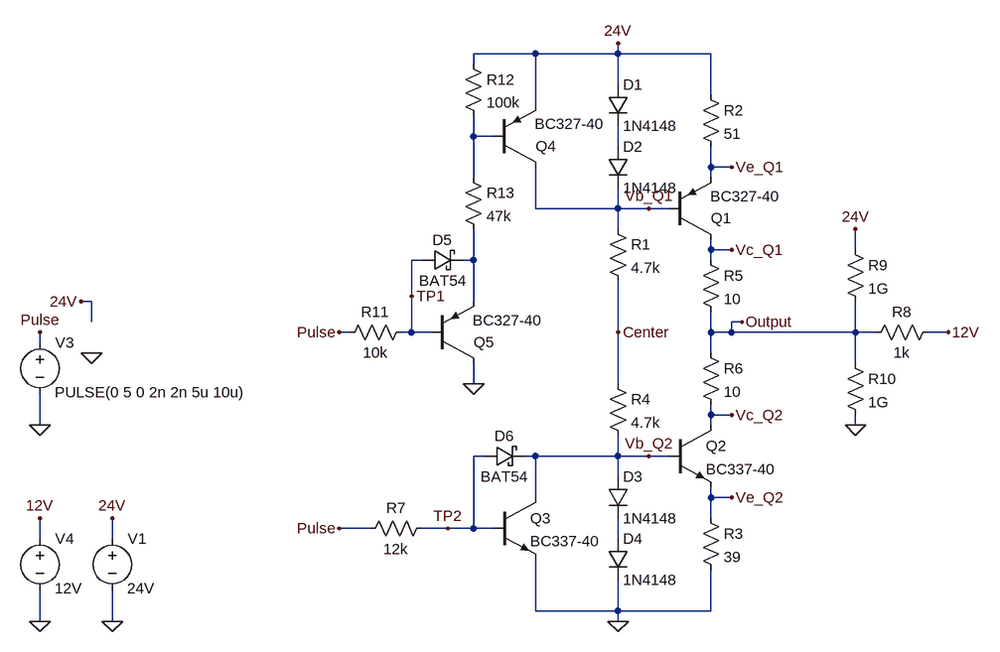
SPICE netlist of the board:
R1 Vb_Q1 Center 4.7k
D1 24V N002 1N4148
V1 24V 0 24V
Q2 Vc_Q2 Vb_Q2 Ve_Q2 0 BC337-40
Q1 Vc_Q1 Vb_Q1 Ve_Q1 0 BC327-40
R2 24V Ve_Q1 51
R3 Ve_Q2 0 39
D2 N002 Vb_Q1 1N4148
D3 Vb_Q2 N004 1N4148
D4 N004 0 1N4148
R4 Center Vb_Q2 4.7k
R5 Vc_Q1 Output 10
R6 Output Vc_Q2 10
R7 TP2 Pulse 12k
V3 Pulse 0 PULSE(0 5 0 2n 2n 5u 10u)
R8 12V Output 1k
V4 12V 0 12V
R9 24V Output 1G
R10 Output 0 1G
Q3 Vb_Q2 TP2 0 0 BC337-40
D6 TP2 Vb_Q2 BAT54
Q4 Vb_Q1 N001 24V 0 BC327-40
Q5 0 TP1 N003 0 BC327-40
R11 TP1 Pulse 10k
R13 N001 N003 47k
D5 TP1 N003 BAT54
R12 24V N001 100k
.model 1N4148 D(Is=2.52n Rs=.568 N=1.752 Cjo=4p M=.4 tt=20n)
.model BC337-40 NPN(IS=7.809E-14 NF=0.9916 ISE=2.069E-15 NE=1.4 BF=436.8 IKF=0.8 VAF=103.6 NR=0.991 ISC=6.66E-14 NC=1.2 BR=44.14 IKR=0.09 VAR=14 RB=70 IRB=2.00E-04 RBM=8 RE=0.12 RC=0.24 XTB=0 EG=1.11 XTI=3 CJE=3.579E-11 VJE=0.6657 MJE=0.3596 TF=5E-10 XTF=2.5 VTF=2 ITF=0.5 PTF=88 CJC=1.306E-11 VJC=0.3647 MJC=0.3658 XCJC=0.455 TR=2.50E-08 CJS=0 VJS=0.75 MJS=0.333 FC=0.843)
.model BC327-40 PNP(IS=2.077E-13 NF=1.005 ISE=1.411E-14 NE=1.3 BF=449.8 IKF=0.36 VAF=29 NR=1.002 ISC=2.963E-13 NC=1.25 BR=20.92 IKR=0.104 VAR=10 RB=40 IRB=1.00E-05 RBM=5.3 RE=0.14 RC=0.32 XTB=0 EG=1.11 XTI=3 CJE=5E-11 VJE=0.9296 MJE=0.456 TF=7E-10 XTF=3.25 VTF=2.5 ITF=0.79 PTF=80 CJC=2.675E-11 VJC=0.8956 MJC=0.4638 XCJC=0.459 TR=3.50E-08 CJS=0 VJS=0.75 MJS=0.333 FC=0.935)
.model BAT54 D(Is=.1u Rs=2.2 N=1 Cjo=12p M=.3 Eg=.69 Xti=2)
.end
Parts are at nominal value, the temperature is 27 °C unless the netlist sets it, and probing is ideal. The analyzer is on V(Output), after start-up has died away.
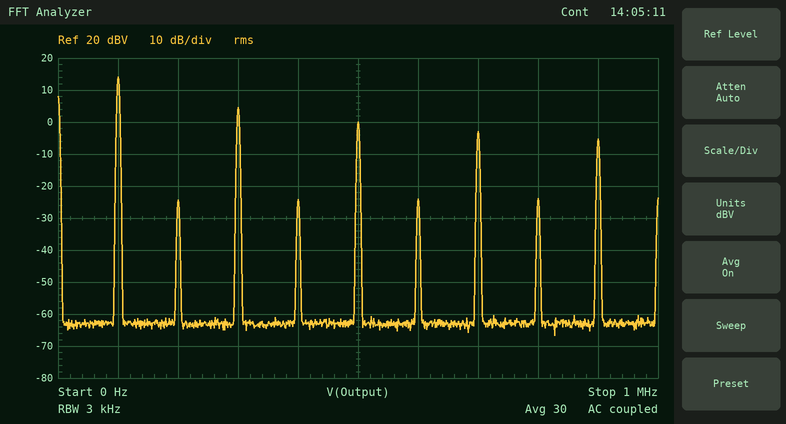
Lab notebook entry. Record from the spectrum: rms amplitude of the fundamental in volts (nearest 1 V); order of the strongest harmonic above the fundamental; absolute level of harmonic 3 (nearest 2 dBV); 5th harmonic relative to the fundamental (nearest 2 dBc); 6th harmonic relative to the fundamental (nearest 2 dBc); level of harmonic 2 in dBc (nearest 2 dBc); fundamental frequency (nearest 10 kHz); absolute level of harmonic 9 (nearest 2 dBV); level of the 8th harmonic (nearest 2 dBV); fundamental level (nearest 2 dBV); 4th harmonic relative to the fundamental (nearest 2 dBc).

5 V
3
4 dBV
-14 dBc
-38 dBc
-38 dBc
100 kHz
-6 dBV
-24 dBV
14 dBV
-38 dBc
